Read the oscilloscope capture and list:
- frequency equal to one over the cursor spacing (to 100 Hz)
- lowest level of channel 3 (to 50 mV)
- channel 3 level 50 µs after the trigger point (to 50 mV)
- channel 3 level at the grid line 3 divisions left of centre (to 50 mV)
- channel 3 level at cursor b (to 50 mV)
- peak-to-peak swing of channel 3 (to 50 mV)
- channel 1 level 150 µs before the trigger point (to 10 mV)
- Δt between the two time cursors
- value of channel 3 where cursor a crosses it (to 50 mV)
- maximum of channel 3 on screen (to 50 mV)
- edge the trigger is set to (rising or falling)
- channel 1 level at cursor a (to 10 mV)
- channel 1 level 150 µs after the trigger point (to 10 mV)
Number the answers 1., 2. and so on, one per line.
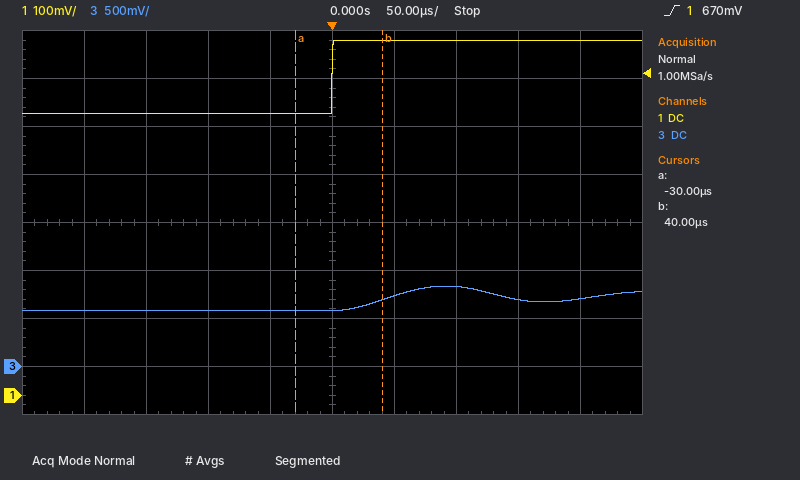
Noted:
1. 14.3 kHz
2. 600 mV
3. 750 mV
4. 600 mV
5. 700 mV
6. 250 mV
7. 590 mV
8. 70 µs
9. 600 mV
10. 850 mV
11. rising
12. 590 mV
13. 740 mV
